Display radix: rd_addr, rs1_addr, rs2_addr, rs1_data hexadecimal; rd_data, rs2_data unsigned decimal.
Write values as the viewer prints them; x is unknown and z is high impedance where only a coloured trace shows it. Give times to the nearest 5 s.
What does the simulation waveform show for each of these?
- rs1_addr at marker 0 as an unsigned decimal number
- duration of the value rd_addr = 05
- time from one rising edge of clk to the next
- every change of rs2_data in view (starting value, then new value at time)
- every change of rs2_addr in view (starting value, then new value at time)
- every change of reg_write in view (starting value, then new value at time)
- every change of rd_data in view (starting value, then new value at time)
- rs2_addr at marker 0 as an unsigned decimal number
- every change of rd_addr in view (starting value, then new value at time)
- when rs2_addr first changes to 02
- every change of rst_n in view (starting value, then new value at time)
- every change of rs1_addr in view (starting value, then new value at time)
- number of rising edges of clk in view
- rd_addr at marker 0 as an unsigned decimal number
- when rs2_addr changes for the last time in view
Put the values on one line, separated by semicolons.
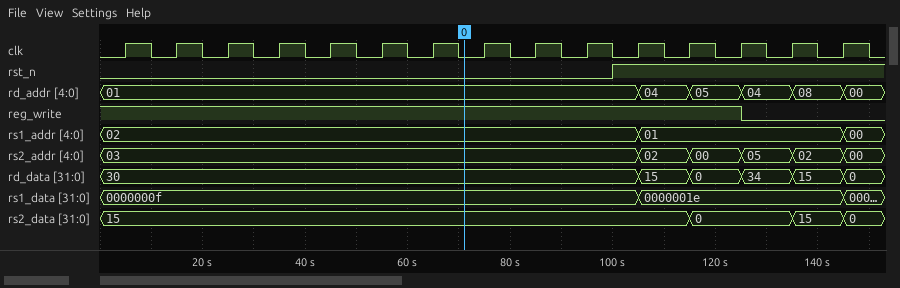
2; 10 s; 10 s; 15, 0 at 115 s, 15 at 135 s, 0 at 145 s; 03, 02 at 105 s, 00 at 115 s, 05 at 125 s, 02 at 135 s, 00 at 145 s; 1, 0 at 125 s; 30, 15 at 105 s, 0 at 115 s, 34 at 125 s, 15 at 135 s, 0 at 145 s; 3; 01, 04 at 105 s, 05 at 115 s, 04 at 125 s, 08 at 135 s, 00 at 145 s; 105 s; 0, 1 at 100 s; 02, 01 at 105 s, 00 at 145 s; 15; 1; 145 s
